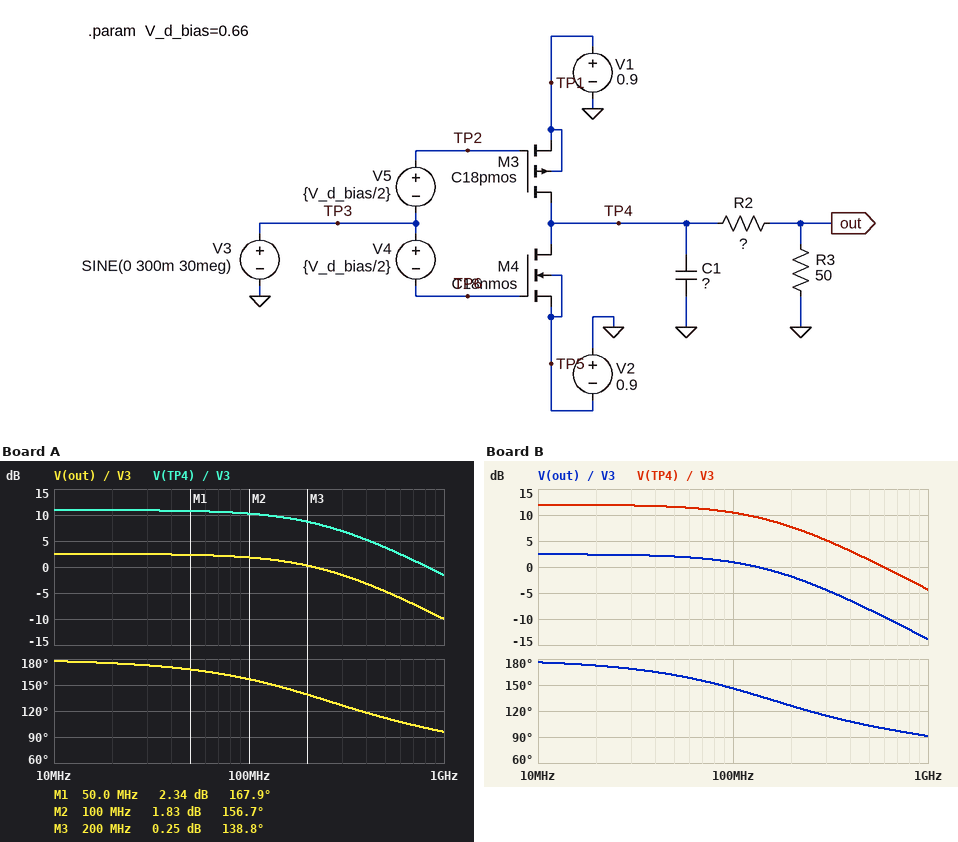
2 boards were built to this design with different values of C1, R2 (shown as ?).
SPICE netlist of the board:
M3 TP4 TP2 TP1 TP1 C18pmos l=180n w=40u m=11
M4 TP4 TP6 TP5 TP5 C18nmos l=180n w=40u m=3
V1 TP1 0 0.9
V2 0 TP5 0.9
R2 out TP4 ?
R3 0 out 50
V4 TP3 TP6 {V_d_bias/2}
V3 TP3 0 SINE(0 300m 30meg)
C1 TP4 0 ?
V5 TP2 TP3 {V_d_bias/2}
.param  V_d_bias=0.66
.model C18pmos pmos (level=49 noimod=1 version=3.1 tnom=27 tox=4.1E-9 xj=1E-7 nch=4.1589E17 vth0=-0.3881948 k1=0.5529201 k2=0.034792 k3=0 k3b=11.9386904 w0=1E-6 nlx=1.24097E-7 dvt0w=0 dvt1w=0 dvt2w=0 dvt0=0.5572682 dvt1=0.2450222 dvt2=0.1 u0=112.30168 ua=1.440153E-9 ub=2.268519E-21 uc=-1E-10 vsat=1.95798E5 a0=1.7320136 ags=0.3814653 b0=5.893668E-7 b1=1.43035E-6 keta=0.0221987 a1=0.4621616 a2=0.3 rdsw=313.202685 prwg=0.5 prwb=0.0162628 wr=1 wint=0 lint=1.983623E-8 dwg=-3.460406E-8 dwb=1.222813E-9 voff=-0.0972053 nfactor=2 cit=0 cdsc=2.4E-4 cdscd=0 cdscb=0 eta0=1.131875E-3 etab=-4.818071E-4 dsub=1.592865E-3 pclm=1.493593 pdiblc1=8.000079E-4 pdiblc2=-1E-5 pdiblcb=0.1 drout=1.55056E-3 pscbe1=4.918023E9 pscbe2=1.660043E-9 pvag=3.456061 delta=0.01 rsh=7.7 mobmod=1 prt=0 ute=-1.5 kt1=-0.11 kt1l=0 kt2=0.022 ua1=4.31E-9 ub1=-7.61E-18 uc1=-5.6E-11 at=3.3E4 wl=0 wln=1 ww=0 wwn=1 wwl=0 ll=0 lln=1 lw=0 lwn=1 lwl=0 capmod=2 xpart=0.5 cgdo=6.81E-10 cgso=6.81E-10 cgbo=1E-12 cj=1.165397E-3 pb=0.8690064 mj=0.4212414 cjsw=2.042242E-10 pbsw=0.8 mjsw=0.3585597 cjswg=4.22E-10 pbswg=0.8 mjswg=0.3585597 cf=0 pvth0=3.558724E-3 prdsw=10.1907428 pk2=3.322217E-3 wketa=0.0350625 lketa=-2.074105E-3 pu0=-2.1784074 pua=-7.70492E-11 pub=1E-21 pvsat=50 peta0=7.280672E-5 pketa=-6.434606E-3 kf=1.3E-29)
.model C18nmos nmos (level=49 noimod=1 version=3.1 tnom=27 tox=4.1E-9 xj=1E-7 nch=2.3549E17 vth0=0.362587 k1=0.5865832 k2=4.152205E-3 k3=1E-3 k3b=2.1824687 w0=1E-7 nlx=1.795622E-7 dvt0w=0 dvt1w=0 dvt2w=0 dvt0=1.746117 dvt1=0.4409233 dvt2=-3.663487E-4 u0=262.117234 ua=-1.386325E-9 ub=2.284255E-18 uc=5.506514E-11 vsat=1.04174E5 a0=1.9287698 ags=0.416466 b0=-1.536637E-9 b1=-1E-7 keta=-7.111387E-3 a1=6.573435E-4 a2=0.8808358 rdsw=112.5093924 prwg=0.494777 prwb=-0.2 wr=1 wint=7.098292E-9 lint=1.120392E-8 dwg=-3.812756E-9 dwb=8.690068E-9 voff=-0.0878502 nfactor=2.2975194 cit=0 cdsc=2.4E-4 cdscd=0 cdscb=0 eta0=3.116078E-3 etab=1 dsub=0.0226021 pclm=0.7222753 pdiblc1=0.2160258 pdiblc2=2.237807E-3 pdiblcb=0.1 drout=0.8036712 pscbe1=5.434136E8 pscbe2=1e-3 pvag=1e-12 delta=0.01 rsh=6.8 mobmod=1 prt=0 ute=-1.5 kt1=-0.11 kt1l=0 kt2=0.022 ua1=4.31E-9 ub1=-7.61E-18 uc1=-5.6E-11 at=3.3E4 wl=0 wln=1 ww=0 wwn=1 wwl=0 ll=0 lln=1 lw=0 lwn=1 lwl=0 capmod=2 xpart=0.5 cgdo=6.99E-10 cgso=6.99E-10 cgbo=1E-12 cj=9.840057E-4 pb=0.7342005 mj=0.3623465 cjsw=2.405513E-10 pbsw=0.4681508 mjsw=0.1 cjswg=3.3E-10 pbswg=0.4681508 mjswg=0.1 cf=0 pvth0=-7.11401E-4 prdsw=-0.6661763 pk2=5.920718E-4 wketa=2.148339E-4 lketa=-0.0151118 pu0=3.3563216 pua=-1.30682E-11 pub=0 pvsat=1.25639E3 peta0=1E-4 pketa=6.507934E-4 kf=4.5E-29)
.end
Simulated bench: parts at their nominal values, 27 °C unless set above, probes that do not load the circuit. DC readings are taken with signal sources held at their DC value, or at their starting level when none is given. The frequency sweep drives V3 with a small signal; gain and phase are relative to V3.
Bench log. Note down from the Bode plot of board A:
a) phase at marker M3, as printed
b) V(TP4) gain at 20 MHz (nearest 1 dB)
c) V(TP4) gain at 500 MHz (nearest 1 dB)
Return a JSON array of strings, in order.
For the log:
["138.8 deg", "11 dB", "4 dB"]
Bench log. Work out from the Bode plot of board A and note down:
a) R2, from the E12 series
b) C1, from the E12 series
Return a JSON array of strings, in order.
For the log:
["82 Ω", "4.7 pF"]
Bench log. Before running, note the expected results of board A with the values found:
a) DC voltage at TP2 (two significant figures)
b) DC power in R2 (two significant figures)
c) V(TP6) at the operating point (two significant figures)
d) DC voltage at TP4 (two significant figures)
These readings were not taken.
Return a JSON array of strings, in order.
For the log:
["330 mV", "400 nW", "-330 mV", "-9.2 mV"]
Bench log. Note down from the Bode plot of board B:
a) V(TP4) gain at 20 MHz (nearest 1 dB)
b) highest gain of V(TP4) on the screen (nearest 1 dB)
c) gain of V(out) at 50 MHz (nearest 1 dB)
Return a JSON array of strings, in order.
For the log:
["12 dB", "12 dB", "2 dB"]
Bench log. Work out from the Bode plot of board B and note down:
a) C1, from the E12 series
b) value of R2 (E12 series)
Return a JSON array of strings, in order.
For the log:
["6.8 pF", "100 Ω"]
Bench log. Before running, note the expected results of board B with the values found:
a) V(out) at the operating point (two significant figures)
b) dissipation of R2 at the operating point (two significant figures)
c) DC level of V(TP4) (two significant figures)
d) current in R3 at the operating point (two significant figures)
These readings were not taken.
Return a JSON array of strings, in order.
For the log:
["-3.5 mV", "480 nW", "-10 mV", "69 µA"]
